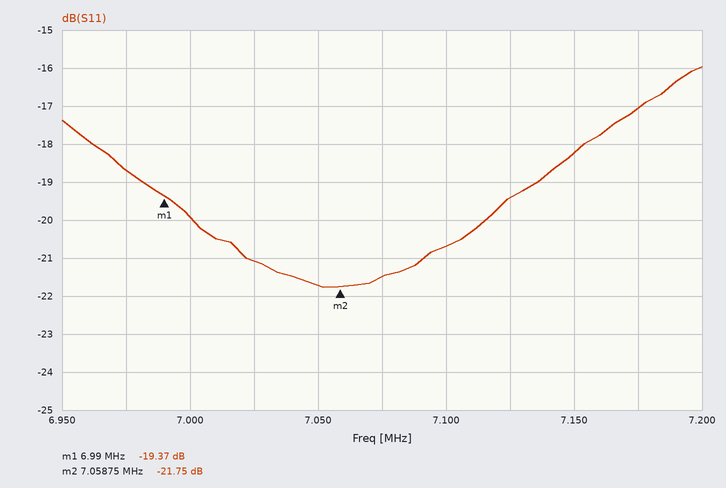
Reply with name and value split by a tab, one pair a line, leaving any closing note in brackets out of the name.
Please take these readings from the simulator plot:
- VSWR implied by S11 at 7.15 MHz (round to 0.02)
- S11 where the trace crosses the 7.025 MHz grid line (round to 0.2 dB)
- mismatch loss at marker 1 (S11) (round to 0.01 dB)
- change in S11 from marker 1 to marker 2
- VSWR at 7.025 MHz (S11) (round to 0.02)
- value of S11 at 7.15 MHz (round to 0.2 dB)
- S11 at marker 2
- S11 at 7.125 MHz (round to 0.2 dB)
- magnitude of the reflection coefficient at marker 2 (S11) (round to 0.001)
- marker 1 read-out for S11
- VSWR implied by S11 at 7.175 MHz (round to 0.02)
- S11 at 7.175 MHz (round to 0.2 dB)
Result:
VSWR implied by S11 at 7.15 MHz	1.28
S11 where the trace crosses the 7.025 MHz grid line	-21.0 dB
mismatch loss at marker 1 (S11)	0.05 dB
change in S11 from marker 1 to marker 2	-2.38 dB
VSWR at 7.025 MHz (S11)	1.20
value of S11 at 7.15 MHz	-18.2 dB
S11 at marker 2	-21.75 dB
S11 at 7.125 MHz	-19.4 dB
magnitude of the reflection coefficient at marker 2 (S11)	0.082
marker 1 read-out for S11	-19.37 dB
VSWR implied by S11 at 7.175 MHz	1.32
S11 at 7.175 MHz	-17.0 dB
